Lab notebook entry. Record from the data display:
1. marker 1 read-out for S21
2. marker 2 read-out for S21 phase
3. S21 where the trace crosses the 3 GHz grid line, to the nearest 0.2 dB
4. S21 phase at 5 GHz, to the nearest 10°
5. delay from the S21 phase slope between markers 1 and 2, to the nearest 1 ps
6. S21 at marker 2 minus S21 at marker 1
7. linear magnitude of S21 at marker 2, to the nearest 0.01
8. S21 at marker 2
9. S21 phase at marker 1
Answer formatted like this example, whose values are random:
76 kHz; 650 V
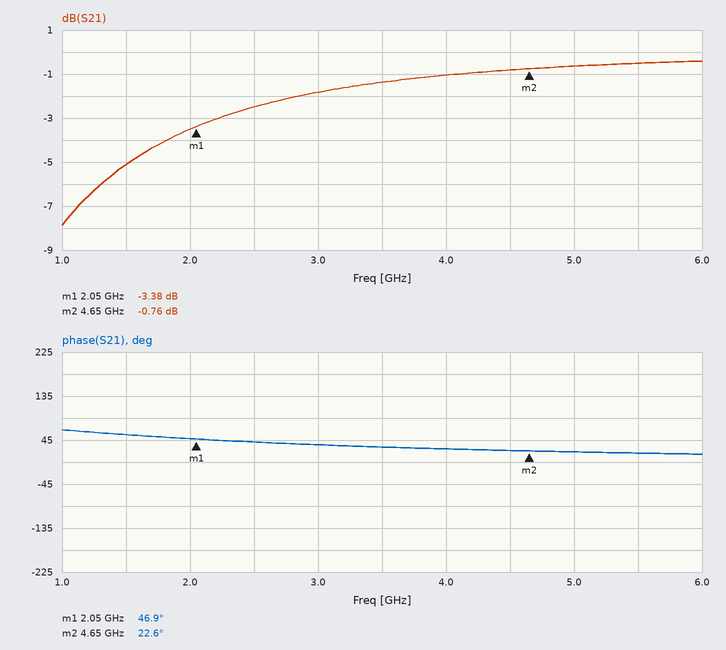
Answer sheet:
-3.38 dB; 22.6°; -1.8 dB; 20°; 26 ps; 2.62 dB; 0.92; -0.76 dB; 46.9°
